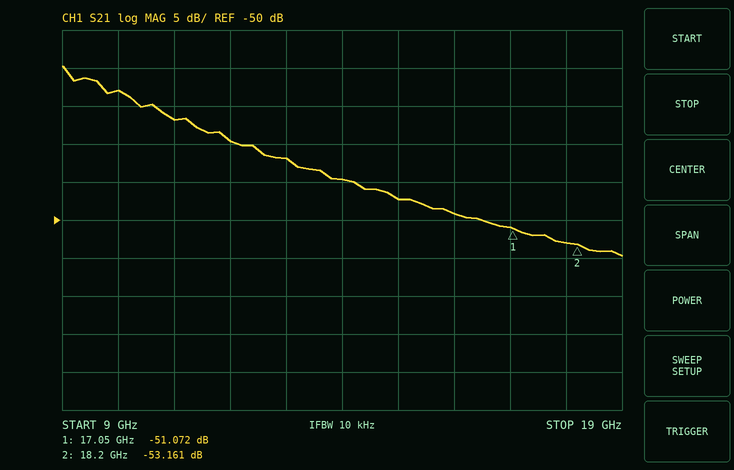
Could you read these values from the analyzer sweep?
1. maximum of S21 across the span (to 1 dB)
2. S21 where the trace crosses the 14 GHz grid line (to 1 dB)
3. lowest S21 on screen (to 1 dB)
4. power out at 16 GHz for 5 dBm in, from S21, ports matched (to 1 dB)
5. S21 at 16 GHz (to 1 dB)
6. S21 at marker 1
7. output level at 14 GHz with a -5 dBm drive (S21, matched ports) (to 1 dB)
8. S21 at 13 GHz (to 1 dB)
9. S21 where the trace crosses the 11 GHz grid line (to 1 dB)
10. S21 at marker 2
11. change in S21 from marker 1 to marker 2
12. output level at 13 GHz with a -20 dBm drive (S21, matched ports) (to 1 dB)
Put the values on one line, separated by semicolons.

-30 dB; -45 dB; -55 dB; -44 dBm; -49 dB; -51.072 dB; -50 dBm; -42 dB; -37 dB; -53.161 dB; -2.089 dB; -62 dBm
